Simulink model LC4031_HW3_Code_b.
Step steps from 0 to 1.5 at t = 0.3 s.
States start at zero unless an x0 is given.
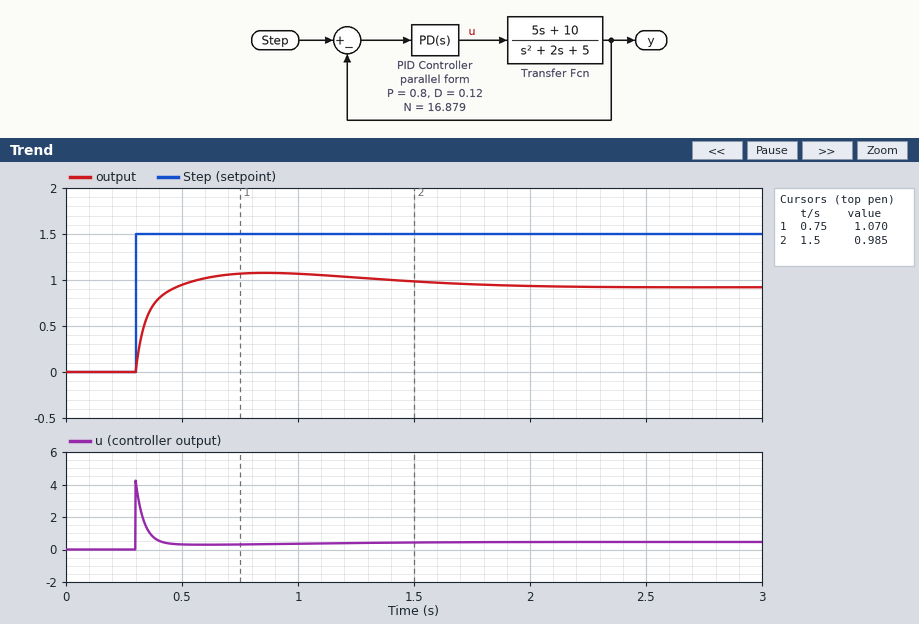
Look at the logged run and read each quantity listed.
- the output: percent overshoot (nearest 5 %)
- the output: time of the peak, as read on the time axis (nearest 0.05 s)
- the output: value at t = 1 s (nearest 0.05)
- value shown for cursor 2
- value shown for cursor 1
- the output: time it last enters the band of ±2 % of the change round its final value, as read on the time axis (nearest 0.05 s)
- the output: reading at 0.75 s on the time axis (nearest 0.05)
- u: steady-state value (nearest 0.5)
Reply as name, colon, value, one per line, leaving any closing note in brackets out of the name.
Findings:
the output: percent overshoot: 15 %
the output: time of the peak, as read on the time axis: 0.85 s
the output: value at t = 1 s: 1.05
value shown for cursor 2: 0.985
value shown for cursor 1: 1.070
the output: time it last enters the band of ±2 % of the change round its final value, as read on the time axis: 1.90 s
the output: reading at 0.75 s on the time axis: 1.05
u: steady-state value: 0.5
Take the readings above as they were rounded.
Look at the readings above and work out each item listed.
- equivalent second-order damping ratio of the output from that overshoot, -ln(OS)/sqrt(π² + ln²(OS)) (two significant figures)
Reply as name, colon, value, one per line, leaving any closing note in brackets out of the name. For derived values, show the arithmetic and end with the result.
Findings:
equivalent second-order damping ratio of the output from that overshoot, -ln(OS)/sqrt(π² + ln²(OS)): ln(0.15) = -1.897; 1.897 / sqrt(9.870 + 3.599) = 0.52
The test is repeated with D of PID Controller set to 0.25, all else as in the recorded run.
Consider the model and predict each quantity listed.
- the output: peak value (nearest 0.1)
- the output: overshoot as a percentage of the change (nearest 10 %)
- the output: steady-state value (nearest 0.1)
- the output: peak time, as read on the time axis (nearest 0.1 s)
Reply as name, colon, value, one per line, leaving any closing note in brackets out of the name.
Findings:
the output: peak value: 1.1
the output: overshoot as a percentage of the change: 20 %
the output: steady-state value: 0.9
the output: peak time, as read on the time axis: 0.8 s
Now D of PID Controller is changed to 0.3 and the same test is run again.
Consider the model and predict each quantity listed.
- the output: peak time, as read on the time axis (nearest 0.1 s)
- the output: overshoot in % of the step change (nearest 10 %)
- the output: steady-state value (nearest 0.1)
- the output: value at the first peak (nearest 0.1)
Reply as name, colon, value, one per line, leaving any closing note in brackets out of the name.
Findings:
the output: peak time, as read on the time axis: 0.7 s
the output: overshoot in % of the step change: 20 %
the output: steady-state value: 0.9
the output: value at the first peak: 1.1
